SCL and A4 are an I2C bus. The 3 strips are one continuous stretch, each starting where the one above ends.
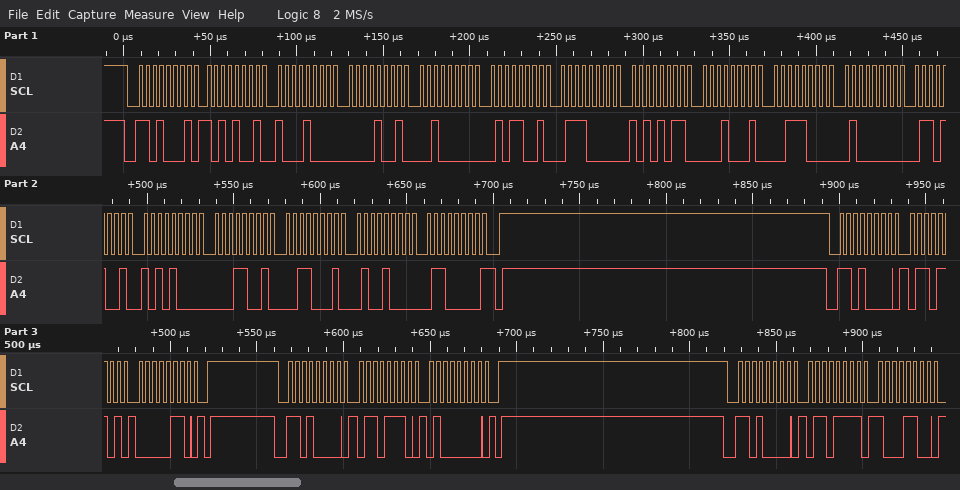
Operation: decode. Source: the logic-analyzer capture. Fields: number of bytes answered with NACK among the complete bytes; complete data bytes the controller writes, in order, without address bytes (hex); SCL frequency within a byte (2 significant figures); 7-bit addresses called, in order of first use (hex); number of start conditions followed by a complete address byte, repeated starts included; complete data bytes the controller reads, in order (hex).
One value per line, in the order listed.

1
6D 06 6E 40 6F 8C
250 kHz
0x68
4
A9 88 09 20 59 70 AB 11 38 40 69 A8 19 31 48 60
